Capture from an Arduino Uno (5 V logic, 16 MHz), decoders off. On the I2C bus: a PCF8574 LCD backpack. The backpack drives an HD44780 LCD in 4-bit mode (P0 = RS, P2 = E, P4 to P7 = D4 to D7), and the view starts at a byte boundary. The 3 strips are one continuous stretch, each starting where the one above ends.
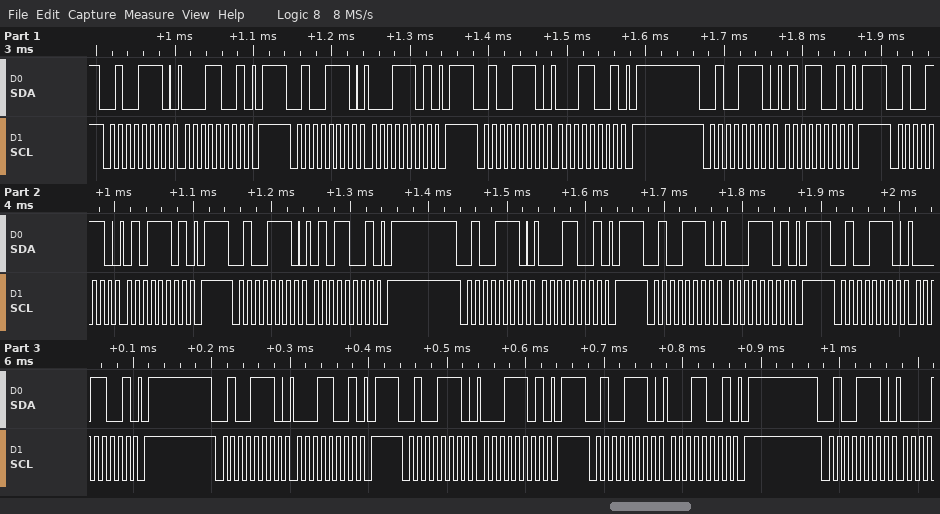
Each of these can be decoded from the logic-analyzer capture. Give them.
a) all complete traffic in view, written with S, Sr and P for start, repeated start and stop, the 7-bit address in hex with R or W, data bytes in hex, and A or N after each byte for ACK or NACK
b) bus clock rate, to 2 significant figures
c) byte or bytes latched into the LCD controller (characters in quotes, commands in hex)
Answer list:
S 27W A 19 A P S 27W A 1D A P S 27W A 19 A P S 27W A 59 A P S 27W A 5D A P S 27W A 59 A P S 27W A 19 A P S 27W A 1D A P S 27W A 19 A P S 27W A 19 A P S 27W A 1D A P S 27W A 19 A P S 27W A
100 kHz
data 0x15 data 0x11
